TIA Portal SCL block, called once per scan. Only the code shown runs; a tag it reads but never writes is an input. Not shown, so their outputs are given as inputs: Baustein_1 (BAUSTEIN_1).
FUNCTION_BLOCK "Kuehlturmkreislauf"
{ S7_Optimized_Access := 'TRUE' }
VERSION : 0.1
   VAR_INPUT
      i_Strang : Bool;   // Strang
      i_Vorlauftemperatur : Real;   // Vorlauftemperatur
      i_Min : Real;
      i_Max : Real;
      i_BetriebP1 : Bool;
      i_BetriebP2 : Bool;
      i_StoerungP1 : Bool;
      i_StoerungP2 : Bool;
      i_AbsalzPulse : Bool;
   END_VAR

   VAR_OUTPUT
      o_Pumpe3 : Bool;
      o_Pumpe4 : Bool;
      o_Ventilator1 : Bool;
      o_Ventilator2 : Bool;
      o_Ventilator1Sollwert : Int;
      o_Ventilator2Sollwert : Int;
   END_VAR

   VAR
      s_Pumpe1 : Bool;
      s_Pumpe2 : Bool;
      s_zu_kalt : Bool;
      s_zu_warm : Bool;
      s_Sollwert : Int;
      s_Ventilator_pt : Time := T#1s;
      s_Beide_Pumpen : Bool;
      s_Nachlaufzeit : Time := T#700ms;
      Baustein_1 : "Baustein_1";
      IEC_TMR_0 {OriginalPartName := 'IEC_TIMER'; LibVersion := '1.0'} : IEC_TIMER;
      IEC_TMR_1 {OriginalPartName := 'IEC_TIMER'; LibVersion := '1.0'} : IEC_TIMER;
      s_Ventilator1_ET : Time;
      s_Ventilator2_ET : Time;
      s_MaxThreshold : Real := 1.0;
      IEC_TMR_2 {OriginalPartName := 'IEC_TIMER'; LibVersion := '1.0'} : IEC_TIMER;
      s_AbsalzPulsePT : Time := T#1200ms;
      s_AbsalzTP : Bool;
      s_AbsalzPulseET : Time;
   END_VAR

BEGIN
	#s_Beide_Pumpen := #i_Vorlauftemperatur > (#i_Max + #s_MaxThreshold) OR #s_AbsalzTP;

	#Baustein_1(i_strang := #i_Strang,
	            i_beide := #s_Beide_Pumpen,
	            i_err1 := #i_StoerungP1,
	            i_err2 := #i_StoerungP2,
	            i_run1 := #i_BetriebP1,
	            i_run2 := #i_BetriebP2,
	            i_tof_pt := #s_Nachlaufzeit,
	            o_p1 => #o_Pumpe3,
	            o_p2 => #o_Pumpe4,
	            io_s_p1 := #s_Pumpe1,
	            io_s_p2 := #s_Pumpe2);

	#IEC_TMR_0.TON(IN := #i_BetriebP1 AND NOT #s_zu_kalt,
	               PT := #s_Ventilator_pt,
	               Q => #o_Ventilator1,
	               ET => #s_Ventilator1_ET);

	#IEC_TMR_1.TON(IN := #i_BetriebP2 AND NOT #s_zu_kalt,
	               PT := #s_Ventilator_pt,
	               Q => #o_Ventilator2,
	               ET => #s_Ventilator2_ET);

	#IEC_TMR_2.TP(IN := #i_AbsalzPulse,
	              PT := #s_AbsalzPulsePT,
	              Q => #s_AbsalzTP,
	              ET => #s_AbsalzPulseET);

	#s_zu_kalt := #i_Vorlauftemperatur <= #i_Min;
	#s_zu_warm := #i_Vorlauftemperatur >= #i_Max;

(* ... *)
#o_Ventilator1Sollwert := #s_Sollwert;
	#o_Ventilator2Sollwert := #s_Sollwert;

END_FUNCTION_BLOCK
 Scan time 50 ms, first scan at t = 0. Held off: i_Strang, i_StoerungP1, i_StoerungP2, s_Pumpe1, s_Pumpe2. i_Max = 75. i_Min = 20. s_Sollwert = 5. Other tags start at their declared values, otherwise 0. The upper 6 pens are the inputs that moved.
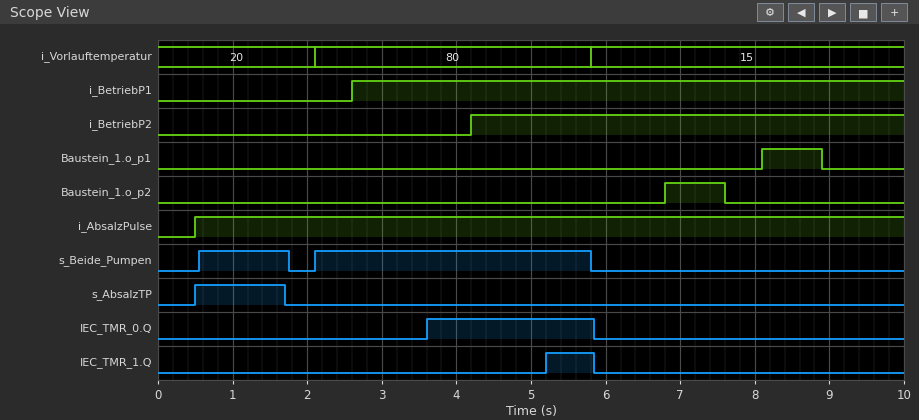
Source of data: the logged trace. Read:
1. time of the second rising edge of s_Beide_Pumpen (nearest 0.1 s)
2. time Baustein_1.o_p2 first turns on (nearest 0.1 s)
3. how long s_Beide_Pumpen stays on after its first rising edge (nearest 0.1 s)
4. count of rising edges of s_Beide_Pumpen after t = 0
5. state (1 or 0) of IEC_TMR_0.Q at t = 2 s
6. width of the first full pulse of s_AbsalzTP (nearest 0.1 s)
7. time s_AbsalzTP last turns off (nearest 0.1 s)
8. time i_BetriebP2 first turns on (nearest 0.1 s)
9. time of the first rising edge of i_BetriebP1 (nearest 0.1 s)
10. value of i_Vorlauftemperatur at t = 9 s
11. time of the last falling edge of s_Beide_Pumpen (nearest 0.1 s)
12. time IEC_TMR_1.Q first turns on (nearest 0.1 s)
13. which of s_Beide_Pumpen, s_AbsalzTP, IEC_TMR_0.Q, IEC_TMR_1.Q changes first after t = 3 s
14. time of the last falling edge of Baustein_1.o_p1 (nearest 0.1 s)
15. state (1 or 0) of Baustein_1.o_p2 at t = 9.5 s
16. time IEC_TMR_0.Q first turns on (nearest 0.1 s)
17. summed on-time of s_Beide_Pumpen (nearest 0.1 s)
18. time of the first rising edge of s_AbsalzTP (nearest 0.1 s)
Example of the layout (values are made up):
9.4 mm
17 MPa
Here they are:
2.1 s
6.8 s
1.2 s
2
0
1.2 s
1.7 s
4.2 s
2.6 s
15
5.8 s
5.2 s
IEC_TMR_0.Q
8.9 s
0
3.6 s
4.9 s
0.5 s
